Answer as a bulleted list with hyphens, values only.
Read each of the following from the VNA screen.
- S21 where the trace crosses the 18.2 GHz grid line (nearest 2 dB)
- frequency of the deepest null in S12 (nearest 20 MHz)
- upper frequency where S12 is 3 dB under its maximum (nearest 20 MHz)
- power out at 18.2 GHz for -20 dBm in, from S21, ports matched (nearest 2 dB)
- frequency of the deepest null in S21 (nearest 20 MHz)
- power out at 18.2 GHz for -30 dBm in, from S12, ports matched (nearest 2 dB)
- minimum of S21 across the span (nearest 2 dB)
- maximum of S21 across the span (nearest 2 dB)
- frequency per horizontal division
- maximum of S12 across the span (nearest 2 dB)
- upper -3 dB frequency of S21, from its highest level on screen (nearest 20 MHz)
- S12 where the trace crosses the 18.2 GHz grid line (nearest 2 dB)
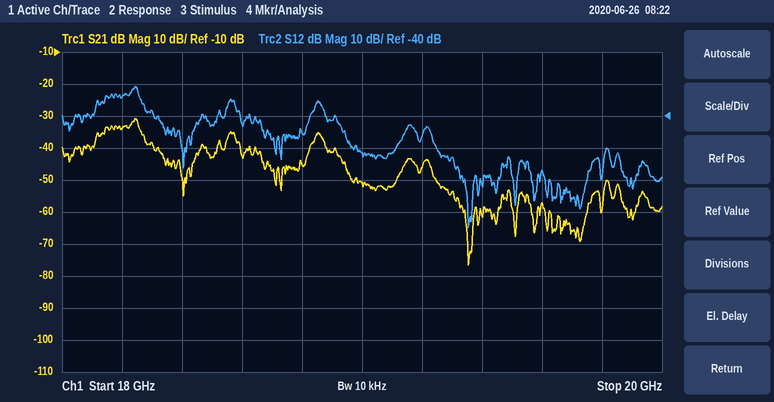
- -34 dB
- 19.36 GHz
- 18.26 GHz
- -54 dBm
- 19.36 GHz
- -64 dBm
- -76 dB
- -30 dB
- 200 MHz
- -30 dB
- 18.26 GHz
- -34 dB
